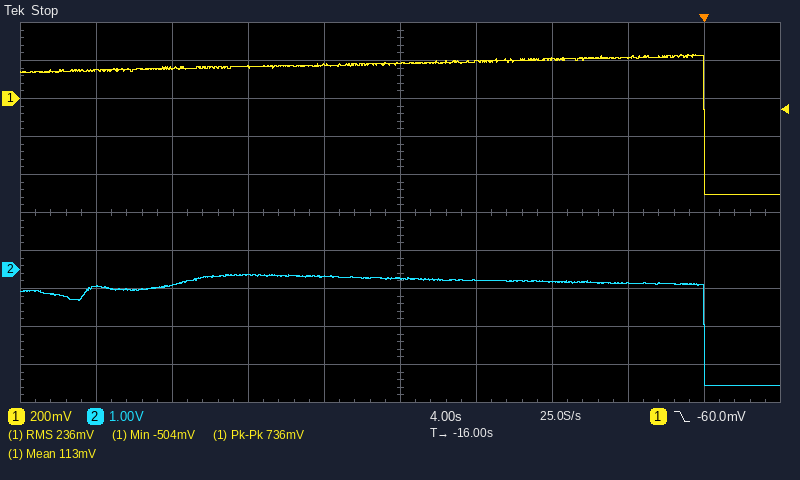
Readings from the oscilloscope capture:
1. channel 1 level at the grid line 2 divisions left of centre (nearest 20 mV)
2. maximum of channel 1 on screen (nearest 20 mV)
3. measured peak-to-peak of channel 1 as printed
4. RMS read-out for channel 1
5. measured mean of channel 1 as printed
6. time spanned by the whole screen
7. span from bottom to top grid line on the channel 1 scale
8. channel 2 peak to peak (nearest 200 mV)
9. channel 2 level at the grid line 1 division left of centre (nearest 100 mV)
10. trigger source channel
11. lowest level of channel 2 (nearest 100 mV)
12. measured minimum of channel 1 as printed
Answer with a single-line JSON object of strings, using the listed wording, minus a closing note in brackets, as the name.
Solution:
{"channel 1 level at the grid line 2 divisions left of centre": "160 mV", "maximum of channel 1 on screen": "240 mV", "measured peak-to-peak of channel 1 as printed": "736 mV", "RMS read-out for channel 1": "236 mV", "measured mean of channel 1 as printed": "113 mV", "time spanned by the whole screen": "40 s", "span from bottom to top grid line on the channel 1 scale": "2 V", "channel 2 peak to peak": "3.0 V", "channel 2 level at the grid line 1 division left of centre": "-200 mV", "trigger source channel": "channel 1", "lowest level of channel 2": "-3.1 V", "measured minimum of channel 1 as printed": "-504 mV"}
